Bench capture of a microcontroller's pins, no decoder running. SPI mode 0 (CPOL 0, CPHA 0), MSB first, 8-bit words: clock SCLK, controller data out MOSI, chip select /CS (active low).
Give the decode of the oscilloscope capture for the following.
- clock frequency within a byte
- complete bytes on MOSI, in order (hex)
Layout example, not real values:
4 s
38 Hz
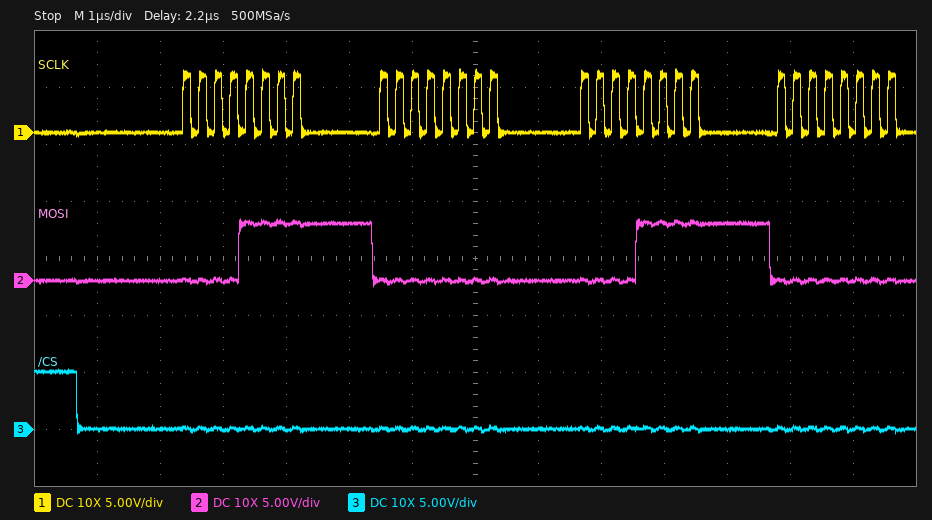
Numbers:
4 MHz
0x0F 0x00 0x0F 0x00
